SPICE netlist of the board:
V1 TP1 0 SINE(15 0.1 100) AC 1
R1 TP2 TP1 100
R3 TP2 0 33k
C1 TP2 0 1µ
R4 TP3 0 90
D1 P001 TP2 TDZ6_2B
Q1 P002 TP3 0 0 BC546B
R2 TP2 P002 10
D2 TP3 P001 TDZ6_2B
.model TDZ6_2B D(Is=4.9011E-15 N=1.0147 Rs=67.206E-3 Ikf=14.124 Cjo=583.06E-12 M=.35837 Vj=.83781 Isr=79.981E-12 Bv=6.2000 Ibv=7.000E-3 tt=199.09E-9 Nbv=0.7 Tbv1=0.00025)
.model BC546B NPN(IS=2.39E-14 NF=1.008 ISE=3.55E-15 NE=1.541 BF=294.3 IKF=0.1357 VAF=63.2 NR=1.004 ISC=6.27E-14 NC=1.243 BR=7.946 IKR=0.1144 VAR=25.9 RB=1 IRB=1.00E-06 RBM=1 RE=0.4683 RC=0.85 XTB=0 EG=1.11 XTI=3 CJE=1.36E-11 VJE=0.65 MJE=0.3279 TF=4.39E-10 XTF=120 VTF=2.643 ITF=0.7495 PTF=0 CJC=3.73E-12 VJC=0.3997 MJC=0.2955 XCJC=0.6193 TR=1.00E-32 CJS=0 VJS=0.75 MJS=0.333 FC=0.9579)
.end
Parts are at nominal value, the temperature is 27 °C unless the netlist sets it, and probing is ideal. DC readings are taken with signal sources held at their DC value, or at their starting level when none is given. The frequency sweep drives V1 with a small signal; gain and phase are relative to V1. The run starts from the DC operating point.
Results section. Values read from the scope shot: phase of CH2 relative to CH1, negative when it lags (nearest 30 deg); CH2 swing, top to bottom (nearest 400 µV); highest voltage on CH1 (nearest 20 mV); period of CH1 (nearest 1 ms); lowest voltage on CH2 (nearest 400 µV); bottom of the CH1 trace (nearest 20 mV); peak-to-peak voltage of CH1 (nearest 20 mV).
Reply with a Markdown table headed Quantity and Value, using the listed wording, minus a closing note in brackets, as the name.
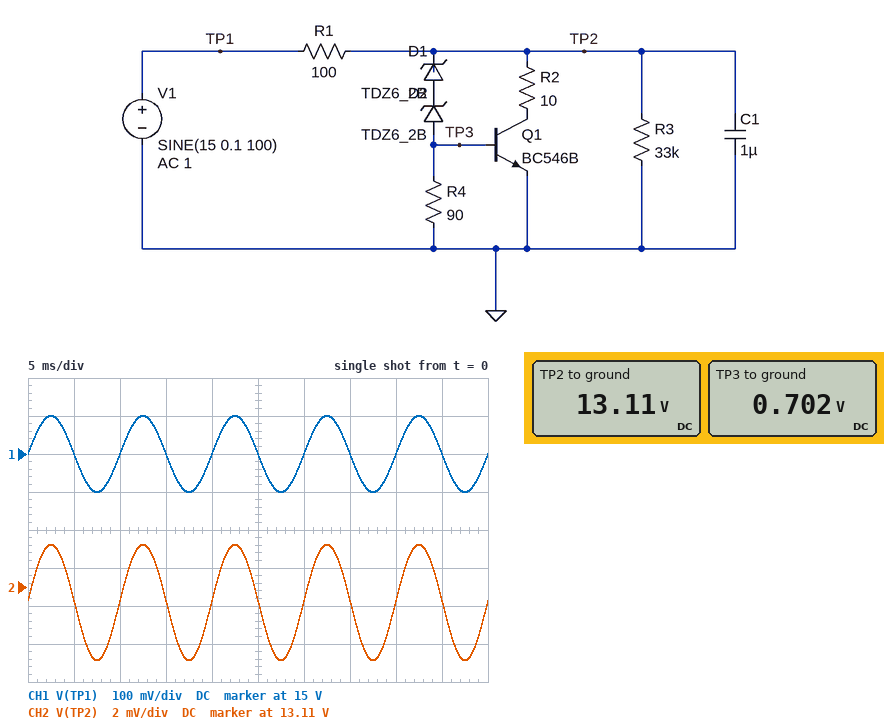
| Quantity | Value |
|---|---|
| phase of CH2 relative to CH1, negative when it lags | 0 deg |
| CH2 swing, top to bottom | 6.0 mV |
| highest voltage on CH1 | 15.10 V |
| period of CH1 | 10 ms |
| lowest voltage on CH2 | 13.1040 V |
| bottom of the CH1 trace | 14.90 V |
| peak-to-peak voltage of CH1 | 200 mV |
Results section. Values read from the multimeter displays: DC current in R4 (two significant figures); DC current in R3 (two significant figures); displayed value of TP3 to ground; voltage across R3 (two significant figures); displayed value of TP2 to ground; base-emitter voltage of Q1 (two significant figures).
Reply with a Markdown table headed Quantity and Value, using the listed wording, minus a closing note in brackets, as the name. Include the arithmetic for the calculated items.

| Quantity | Value |
|---|---|
| DC current in R4 | (702 mV) / 90 Ω = 7.8 mA |
| DC current in R3 | (13.11 V) / 33 kΩ = 400 µA |
| displayed value of TP3 to ground | 0.702 V |
| voltage across R3 | 13.11 V = 13 V |
| displayed value of TP2 to ground | 13.11 V |
| base-emitter voltage of Q1 | 702 mV = 700 mV |
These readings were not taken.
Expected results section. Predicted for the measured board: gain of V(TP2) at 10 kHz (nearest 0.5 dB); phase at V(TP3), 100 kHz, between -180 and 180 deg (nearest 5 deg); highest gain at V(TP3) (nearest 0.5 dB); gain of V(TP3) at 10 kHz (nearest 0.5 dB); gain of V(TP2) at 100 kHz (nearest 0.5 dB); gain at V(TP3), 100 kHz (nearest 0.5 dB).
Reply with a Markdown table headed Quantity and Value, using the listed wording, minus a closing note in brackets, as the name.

| Quantity | Value |
|---|---|
| gain of V(TP2) at 10 kHz | -30.5 dB |
| phase at V(TP3), 100 kHz, between -180 and 180 deg | -60 deg |
| highest gain at V(TP3) | -31.0 dB |
| gain of V(TP3) at 10 kHz | -31.0 dB |
| gain of V(TP2) at 100 kHz | -37.0 dB |
| gain at V(TP3), 100 kHz | -37.5 dB |
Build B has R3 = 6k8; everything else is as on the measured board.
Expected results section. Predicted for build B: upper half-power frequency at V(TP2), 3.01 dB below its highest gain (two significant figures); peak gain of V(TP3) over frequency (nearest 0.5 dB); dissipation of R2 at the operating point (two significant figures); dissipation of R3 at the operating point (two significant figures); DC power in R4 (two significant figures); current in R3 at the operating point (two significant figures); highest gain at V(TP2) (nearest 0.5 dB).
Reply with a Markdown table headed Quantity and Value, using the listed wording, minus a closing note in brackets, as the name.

| Quantity | Value |
|---|---|
| upper half-power frequency at V(TP2), 3.01 dB below its highest gain | 47 kHz |
| peak gain of V(TP3) over frequency | -30.0 dB |
| dissipation of R2 at the operating point | 860 µW |
| dissipation of R3 at the operating point | 25 mW |
| DC power in R4 | 5.4 mW |
| current in R3 at the operating point | 1.9 mA |
| highest gain at V(TP2) | -29.5 dB |
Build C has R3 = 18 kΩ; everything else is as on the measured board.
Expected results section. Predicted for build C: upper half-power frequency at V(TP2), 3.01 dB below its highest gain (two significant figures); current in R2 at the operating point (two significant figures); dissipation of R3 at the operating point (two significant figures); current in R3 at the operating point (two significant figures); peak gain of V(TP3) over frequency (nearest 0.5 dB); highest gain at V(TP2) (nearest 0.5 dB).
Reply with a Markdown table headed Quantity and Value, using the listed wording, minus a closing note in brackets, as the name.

| Quantity | Value |
|---|---|
| upper half-power frequency at V(TP2), 3.01 dB below its highest gain | 51 kHz |
| current in R2 at the operating point | 10 mA |
| dissipation of R3 at the operating point | 9.5 mW |
| current in R3 at the operating point | 730 µA |
| peak gain of V(TP3) over frequency | -30.5 dB |
| highest gain at V(TP2) | -30.0 dB |
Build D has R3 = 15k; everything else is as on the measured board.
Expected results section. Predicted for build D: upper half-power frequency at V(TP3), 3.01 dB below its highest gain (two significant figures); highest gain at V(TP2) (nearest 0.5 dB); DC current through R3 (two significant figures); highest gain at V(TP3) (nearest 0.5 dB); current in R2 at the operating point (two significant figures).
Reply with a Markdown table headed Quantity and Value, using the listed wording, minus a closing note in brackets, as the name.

| Quantity | Value |
|---|---|
| upper half-power frequency at V(TP3), 3.01 dB below its highest gain | 51 kHz |
| highest gain at V(TP2) | -30.0 dB |
| DC current through R3 | 870 µA |
| highest gain at V(TP3) | -30.5 dB |
| current in R2 at the operating point | 10 mA |
